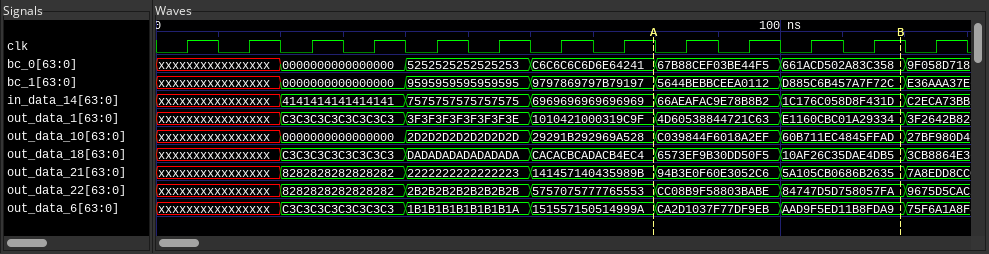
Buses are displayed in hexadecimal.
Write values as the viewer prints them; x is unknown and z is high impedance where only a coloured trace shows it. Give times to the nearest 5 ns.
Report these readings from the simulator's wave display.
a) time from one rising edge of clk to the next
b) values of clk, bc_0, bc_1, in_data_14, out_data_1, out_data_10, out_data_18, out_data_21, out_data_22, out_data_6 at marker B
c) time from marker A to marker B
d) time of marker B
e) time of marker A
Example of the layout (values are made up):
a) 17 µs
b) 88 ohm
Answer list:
a) 10 ns
b) clk=1, bc_0=661ACD502A83C358, bc_1=D885C6B457A7F72C, in_data_14=1C176C058D8F431D, out_data_1=E1160CBC01A29334, out_data_10=60B711EC4845FFAD, out_data_18=10AF26C35DAE4DB5, out_data_21=5A105CB0686B2635, out_data_22=84747D5D758057FA, out_data_6=AAD9F5ED11B8FDA9
c) 40 ns
d) 120 ns
e) 80 ns
